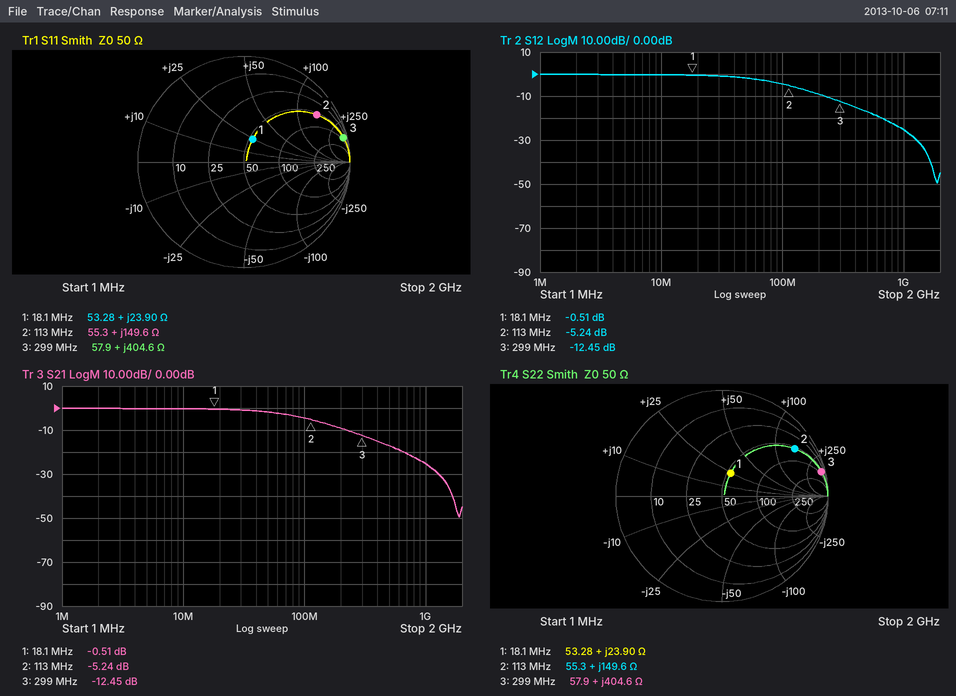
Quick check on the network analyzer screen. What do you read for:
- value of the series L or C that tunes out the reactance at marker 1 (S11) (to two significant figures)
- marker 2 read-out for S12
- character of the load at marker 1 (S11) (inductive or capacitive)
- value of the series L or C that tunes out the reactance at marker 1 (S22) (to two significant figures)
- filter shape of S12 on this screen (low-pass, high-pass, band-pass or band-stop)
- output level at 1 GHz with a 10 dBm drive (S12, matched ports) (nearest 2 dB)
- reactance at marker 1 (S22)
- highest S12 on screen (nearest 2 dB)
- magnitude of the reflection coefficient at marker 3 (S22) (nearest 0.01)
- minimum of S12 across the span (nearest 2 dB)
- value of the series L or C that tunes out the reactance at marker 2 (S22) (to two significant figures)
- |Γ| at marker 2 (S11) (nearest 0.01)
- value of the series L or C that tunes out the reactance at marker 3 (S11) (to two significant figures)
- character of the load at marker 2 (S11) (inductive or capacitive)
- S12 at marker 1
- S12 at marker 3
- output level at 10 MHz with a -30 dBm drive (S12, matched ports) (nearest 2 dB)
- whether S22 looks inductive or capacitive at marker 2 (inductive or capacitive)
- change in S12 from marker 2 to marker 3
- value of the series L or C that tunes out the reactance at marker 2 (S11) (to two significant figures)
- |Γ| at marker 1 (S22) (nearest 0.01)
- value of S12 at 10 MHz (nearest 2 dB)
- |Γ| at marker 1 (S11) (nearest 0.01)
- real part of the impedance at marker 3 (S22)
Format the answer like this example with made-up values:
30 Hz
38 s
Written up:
370 pF
-5.24 dB
inductive
370 pF
low-pass
-16 dBm
+23.90 Ω
0 dB
0.97
-50 dB
9.4 pF
0.82
1.3 pF
inductive
-0.51 dB
-12.45 dB
-30 dBm
inductive
-7.21 dB
9.4 pF
0.23
0 dB
0.23
57.9 Ω
